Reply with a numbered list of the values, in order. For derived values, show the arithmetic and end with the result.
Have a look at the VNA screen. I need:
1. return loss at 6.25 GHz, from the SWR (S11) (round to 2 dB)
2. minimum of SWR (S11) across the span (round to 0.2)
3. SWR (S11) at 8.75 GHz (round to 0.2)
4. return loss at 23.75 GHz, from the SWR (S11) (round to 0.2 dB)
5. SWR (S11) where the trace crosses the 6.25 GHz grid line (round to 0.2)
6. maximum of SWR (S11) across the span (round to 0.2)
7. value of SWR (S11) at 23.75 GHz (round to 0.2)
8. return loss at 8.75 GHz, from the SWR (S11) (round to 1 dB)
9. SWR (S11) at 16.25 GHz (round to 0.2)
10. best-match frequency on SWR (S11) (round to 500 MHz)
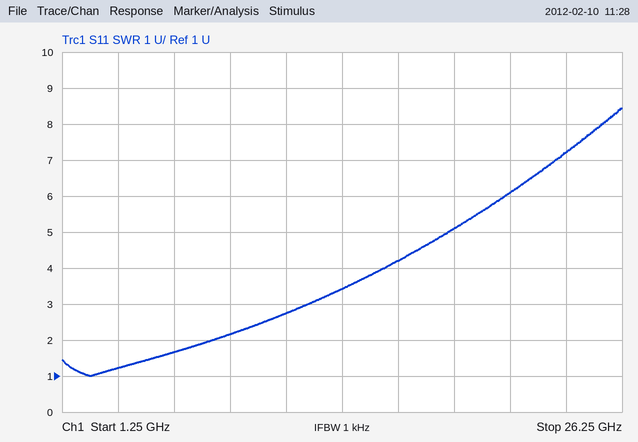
1. −20 log10((1.6 − 1)/(1.6 + 1)) ≈ 12.7 dB, so 12 dB to the nearest 2 dB
2. 1.0
3. 2.2
4. −20 log10((7.2 − 1)/(7.2 + 1)) ≈ 2.4 dB
5. 1.6
6. 8.4
7. 7.2
8. −20 log10((2.2 − 1)/(2.2 + 1)) ≈ 9 dB
9. 4.2
10. 2.5 GHz
